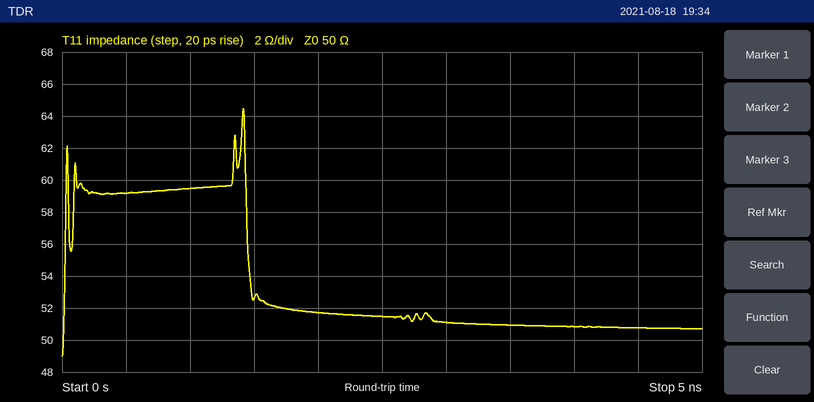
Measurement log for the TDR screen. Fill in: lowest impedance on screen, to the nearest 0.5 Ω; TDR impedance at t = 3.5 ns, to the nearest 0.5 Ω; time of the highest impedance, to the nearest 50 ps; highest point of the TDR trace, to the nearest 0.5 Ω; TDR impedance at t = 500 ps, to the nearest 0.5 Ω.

49.0 Ω
51.0 Ω
1.40 ns
64.5 Ω
59.0 Ω
